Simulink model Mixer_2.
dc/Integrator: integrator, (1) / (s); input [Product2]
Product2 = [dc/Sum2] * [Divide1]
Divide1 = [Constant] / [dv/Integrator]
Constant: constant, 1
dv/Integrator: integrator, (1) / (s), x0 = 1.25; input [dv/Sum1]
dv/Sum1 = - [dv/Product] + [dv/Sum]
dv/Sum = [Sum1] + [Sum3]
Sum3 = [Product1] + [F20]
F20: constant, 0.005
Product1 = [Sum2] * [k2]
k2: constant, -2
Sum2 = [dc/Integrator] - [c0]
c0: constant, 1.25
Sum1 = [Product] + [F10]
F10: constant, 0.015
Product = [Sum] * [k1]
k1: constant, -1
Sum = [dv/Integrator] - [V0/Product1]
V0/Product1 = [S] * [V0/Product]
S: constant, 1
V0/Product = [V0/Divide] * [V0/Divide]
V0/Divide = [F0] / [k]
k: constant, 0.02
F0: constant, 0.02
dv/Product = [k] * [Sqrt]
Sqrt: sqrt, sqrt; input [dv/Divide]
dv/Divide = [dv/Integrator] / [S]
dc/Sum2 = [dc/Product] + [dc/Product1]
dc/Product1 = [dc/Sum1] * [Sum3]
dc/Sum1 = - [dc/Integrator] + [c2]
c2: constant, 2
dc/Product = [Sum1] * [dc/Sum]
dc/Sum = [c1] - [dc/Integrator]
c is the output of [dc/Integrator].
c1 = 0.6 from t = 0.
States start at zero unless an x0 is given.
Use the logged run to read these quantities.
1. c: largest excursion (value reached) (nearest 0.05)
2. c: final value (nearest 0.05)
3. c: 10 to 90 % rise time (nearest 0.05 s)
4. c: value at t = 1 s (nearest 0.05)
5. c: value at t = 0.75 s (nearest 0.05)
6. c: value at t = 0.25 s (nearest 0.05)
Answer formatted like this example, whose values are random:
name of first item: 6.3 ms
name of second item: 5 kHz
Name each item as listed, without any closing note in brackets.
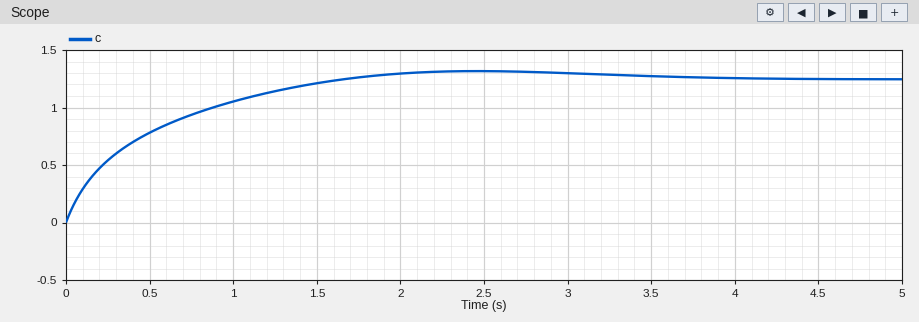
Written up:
c: largest excursion (value reached): 1.30
c: final value: 1.25
c: 10 to 90 % rise time: 1.15 s
c: value at t = 1 s: 1.05
c: value at t = 0.75 s: 0.95
c: value at t = 0.25 s: 0.55
